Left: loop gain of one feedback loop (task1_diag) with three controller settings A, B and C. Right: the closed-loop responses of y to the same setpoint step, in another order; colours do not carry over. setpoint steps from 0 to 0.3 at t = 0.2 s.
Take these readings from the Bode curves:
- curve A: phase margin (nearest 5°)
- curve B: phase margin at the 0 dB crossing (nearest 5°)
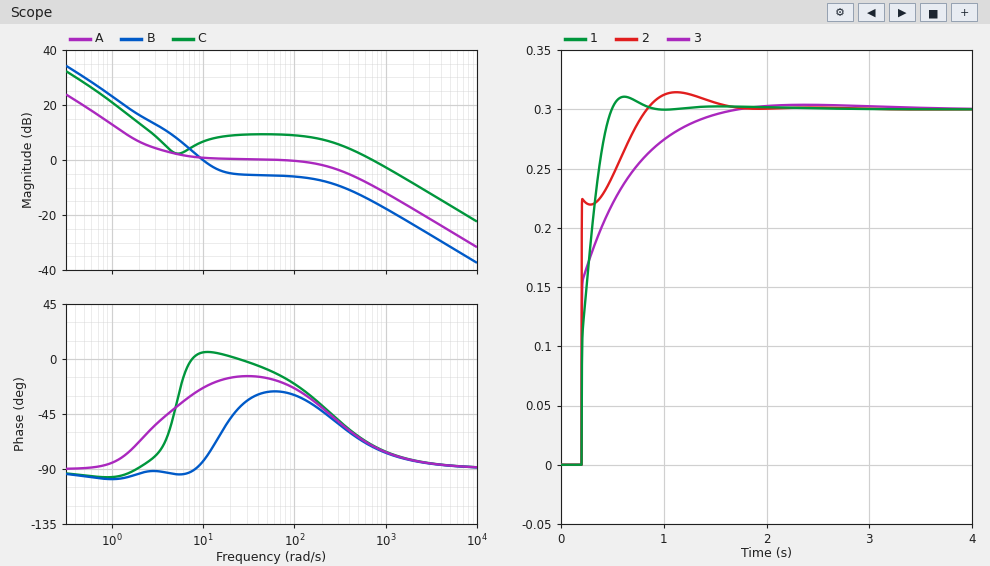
160°
95°
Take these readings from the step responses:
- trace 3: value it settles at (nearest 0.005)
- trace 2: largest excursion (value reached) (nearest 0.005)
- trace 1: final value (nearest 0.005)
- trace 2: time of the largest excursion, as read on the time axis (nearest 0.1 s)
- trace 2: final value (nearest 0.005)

0.300
0.315
0.300
1.1 s
0.300
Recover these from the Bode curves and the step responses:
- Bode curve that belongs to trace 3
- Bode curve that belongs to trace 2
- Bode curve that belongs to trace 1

A
C
B
